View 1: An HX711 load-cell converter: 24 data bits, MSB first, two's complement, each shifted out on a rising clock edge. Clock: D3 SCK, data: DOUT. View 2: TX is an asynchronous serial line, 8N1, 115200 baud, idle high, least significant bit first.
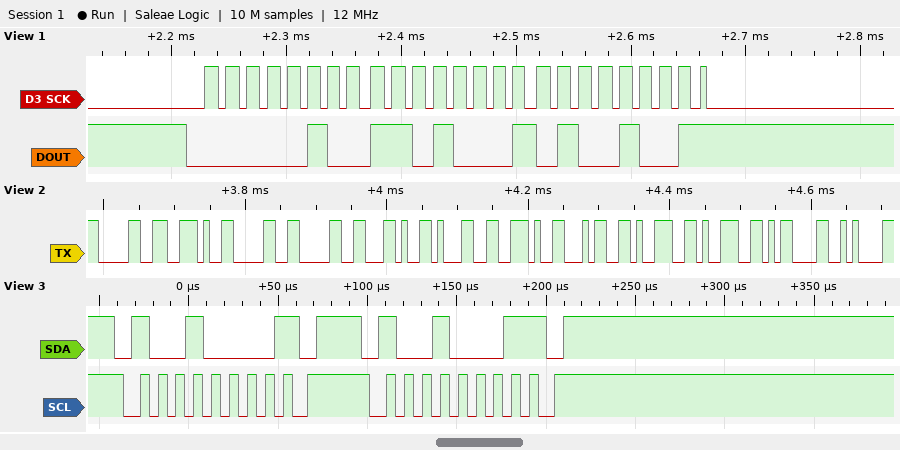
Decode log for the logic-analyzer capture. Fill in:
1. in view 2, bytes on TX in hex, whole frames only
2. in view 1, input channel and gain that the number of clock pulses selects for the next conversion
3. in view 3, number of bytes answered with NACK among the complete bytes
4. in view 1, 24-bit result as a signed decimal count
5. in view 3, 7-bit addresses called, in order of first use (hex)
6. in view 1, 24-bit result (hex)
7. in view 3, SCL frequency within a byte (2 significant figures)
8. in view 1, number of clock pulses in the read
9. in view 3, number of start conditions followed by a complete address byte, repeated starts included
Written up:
0x30 0x2E 0x30 0x30 0x2C 0x31 0x2E 0x34 0x39 0x39 0x0D 0x0A
channel A, gain 128
2
315721
0x48
0x04D149
100 kHz
25
2
